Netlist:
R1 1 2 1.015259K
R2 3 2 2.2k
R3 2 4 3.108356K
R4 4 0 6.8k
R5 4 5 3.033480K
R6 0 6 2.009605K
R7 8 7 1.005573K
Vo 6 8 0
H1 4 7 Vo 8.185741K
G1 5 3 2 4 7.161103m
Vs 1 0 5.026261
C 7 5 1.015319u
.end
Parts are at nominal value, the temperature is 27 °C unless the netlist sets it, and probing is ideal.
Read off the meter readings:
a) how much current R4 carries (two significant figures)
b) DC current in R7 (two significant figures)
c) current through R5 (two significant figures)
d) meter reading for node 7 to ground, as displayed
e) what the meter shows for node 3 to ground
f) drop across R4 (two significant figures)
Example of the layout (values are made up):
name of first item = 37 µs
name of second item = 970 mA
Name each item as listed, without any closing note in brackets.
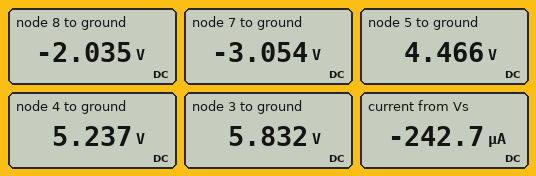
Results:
how much current R4 carries = 770 µA
DC current in R7 = 1.0 mA
current through R5 = 250 µA
meter reading for node 7 to ground, as displayed = -3.054 V
what the meter shows for node 3 to ground = 5.832 V
drop across R4 = 5.2 V
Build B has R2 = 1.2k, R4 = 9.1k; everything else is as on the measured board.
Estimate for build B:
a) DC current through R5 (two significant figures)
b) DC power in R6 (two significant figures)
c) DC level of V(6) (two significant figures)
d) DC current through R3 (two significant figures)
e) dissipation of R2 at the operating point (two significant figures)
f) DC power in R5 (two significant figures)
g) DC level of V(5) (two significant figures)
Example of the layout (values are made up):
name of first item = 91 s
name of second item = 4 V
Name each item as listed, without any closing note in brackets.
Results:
DC current through R5 = 470 µA
DC power in R6 = 2.2 mW
DC level of V(6) = -2.1 V
DC current through R3 = 21 µA
dissipation of R2 at the operating point = 270 µW
DC power in R5 = 680 µW
DC level of V(5) = 4.0 V
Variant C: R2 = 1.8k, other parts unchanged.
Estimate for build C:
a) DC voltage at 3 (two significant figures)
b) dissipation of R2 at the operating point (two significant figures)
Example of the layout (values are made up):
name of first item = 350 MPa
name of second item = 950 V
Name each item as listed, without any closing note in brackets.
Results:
DC voltage at 3 = 5.7 V
dissipation of R2 at the operating point = 120 µW
